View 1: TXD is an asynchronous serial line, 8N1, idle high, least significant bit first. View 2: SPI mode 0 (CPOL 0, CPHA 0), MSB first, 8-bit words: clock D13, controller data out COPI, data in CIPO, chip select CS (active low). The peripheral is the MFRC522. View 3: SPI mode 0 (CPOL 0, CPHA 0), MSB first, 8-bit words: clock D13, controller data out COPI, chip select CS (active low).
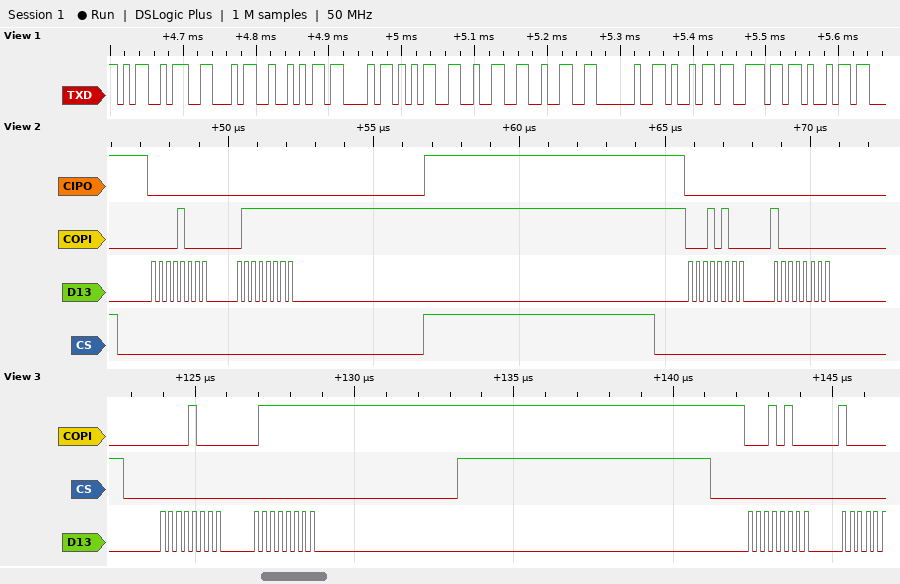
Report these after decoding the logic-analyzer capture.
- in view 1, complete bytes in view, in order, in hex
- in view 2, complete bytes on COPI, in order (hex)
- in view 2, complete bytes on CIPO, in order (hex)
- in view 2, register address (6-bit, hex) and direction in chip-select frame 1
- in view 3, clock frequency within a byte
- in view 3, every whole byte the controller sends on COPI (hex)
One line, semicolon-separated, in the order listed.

0x4D 0x46 0x52 0x43 0x35 0x32 0x32 0x20 0x69 0x6E 0x69; 08 7F 14 80; 00 00 00 00; 0x04 write; 4 MHz; 08 7F 14
